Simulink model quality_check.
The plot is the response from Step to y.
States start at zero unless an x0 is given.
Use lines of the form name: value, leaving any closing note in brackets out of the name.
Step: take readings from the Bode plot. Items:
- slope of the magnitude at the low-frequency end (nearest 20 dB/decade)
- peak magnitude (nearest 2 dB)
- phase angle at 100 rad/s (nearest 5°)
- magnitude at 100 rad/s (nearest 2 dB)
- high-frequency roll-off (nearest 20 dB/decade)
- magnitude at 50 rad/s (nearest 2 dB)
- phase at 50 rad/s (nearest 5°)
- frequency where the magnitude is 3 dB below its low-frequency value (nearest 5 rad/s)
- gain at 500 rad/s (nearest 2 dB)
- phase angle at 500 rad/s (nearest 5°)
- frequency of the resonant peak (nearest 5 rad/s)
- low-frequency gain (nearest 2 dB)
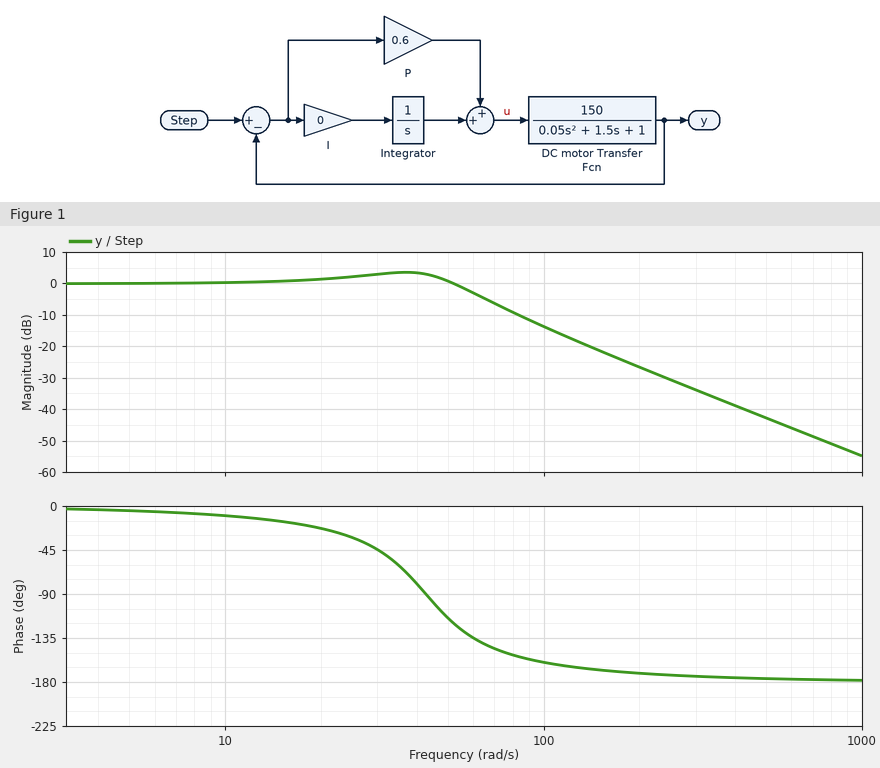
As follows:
slope of the magnitude at the low-frequency end: 0 dB/decade
peak magnitude: 4 dB
phase angle at 100 rad/s: -160°
magnitude at 100 rad/s: -14 dB
high-frequency roll-off: -40 dB/decade
magnitude at 50 rad/s: 0 dB
phase at 50 rad/s: -115°
frequency where the magnitude is 3 dB below its low-frequency value: 60 rad/s
gain at 500 rad/s: -42 dB
phase angle at 500 rad/s: -175°
frequency of the resonant peak: 35 rad/s
low-frequency gain: 0 dB
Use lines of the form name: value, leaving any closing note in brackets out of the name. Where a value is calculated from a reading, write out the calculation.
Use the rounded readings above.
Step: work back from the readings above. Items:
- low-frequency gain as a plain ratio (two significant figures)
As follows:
low-frequency gain as a plain ratio: 10^(0 / 20) = 1.0
